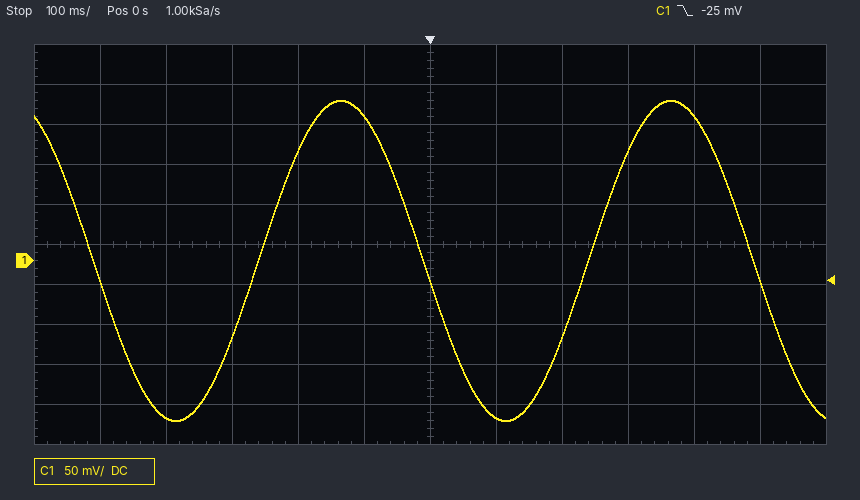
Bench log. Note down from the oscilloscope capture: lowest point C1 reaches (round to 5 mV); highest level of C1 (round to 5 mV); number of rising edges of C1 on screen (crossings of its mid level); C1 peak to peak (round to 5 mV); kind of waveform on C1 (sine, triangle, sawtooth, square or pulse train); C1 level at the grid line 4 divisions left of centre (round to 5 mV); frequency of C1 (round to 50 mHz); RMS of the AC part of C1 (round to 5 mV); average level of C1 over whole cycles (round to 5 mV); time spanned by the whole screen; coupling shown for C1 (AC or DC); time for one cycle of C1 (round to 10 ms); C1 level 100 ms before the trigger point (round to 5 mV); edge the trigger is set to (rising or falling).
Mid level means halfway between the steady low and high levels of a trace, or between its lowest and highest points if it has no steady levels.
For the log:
-200 mV
200 mV
2
400 mV
sine
-195 mV
2.00 Hz
140 mV
0 mV
1.2 s
DC
500 ms
180 mV
falling
